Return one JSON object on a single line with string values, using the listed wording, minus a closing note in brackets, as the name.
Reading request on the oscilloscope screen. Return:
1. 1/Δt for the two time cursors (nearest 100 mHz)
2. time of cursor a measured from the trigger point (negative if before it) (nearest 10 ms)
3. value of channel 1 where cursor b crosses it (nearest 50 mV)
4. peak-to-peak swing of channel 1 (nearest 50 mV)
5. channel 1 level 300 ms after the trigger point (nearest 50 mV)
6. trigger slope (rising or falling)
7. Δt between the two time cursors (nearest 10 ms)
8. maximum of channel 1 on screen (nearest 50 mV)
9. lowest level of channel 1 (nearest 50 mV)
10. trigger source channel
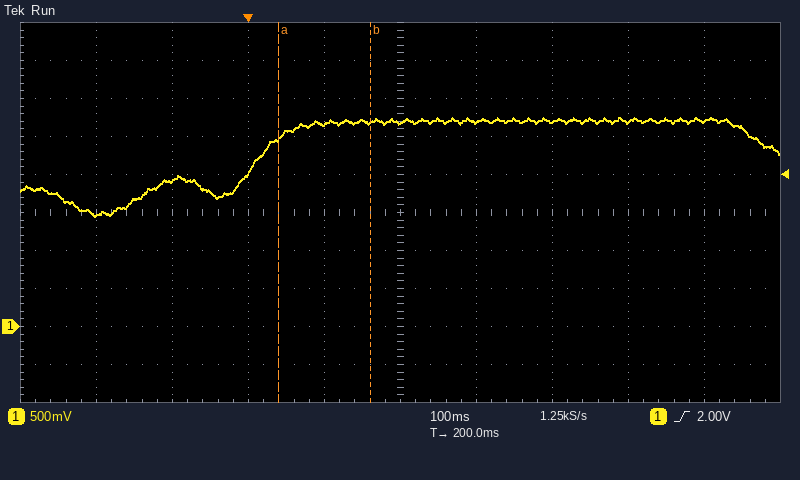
{"1/Δt for the two time cursors": "8.3 Hz", "time of cursor a measured from the trigger point (negative if before it)": "+40 ms", "value of channel 1 where cursor b crosses it": "2.70 V", "peak-to-peak swing of channel 1": "1.30 V", "channel 1 level 300 ms after the trigger point": "2.70 V", "trigger slope": "rising", "Δt between the two time cursors": "120 ms", "maximum of channel 1 on screen": "2.75 V", "lowest level of channel 1": "1.45 V", "trigger source channel": "channel 1"}
